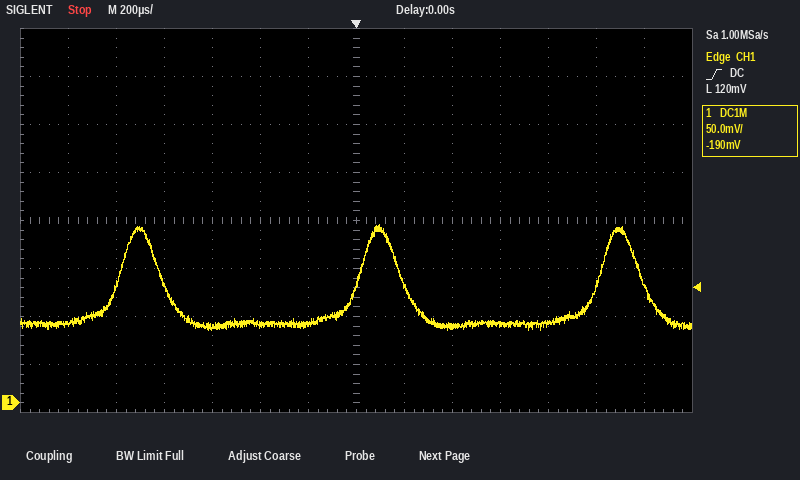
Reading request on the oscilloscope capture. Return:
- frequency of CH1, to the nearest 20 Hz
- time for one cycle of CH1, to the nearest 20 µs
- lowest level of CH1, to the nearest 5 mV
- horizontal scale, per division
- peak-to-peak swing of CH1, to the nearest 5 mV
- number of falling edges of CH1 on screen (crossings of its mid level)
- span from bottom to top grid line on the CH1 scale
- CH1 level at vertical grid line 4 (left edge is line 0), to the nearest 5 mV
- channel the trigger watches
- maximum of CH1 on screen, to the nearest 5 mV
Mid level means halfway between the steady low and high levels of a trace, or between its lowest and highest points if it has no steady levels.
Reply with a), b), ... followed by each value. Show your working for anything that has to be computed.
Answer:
a) 1 / 1.00 ms ≈ 1.00 kHz
b) 1.00 ms
c) 75 mV
d) 200 µs
e) 185 mV − (75 mV) = 110 mV
f) 3
g) 400 mV
h) 80 mV
i) CH1
j) 185 mV
